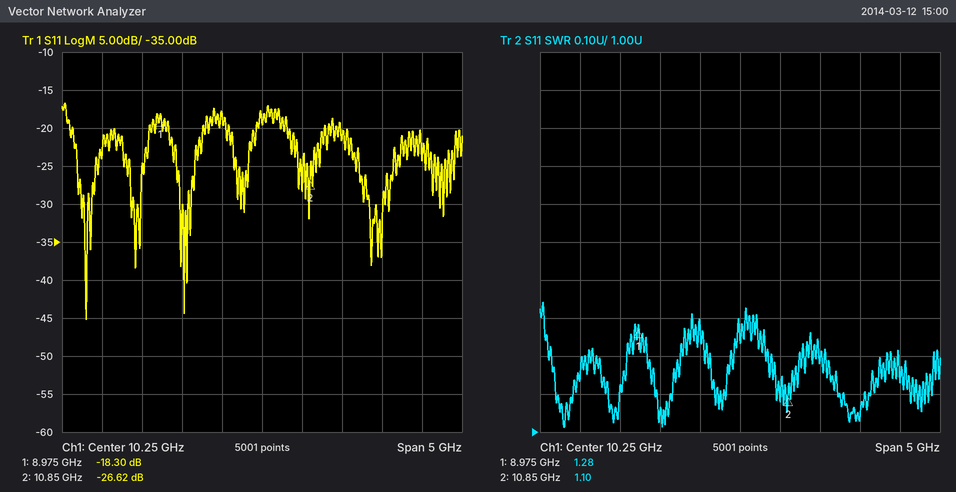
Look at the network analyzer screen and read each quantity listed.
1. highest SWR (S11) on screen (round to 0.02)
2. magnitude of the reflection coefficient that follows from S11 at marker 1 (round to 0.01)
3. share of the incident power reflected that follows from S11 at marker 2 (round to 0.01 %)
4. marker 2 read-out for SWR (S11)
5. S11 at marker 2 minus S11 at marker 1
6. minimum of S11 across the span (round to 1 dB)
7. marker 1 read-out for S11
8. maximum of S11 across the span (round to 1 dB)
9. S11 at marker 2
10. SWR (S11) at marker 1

1.34
0.12
0.22 %
1.10
-8.32 dB
-45 dB
-18.30 dB
-17 dB
-26.62 dB
1.28
